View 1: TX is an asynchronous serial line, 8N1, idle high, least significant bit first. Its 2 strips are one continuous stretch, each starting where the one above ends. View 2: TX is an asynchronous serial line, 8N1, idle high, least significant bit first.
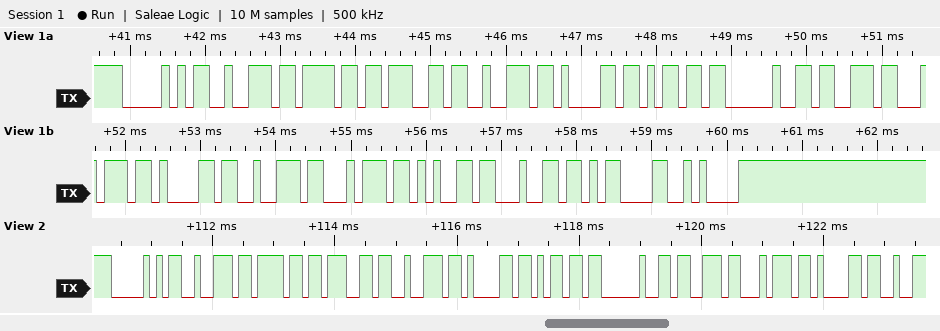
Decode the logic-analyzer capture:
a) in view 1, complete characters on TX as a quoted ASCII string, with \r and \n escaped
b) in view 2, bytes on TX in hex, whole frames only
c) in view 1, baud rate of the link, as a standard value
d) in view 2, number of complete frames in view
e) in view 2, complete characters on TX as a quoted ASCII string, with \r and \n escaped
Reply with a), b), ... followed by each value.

a) "Program started\r\n"
b) 50 72 6F 67 72 61 6D 20 73 74 61
c) 9600 baud
d) 11
e) "Program sta"
